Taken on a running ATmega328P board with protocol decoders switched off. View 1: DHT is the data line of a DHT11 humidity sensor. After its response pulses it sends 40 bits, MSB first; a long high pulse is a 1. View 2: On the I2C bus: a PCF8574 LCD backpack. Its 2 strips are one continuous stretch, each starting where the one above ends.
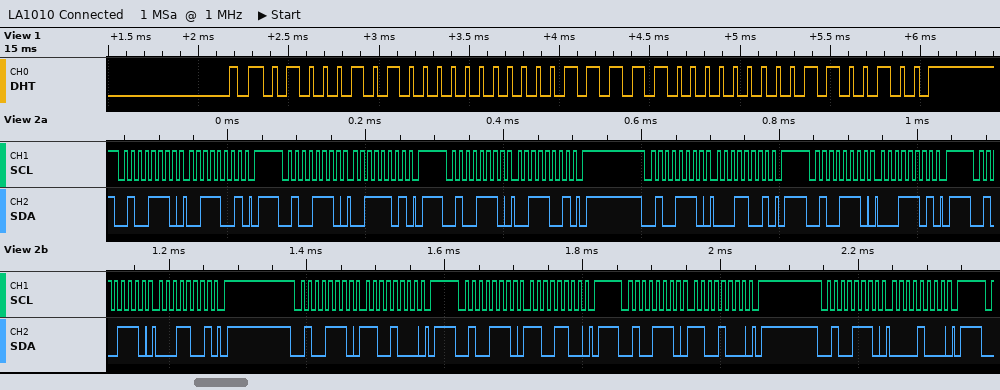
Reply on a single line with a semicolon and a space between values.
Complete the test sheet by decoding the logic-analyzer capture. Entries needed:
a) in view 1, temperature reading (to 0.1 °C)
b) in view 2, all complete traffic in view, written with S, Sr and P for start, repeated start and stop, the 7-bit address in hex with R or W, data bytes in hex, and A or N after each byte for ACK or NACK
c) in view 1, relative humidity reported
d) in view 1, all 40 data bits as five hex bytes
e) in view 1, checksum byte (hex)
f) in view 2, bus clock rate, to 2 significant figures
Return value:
31.0 °C; S 27W A 39 A P S 27W A 3D A P S 27W A 39 A P S 27W A 19 A P S 27W A 1D A P S 27W A 19 A P S 27W A C8 A P S 27W A CC A P S 27W A C8 A P S 27W A 08 A P; 69 %; 45 00 1F 00 64; 0x64; 100 kHz
